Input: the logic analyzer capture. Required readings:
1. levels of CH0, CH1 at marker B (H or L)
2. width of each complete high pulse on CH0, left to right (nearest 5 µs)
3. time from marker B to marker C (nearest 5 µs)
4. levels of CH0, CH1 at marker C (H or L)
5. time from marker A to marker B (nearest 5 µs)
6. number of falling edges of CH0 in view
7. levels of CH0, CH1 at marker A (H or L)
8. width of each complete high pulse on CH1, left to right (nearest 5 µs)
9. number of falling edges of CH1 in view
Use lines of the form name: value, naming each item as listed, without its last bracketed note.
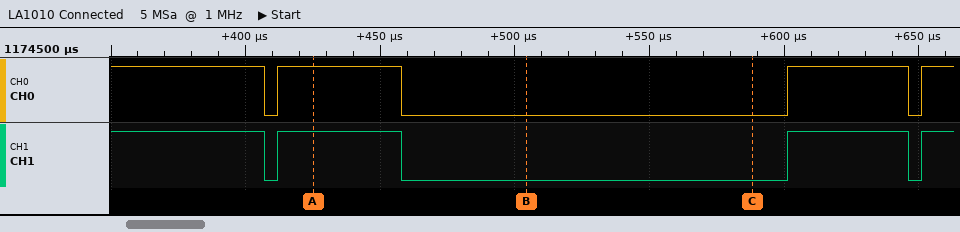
levels of CH0, CH1 at marker B: CH0=L, CH1=L
width of each complete high pulse on CH0, left to right: 45 µs, 45 µs
time from marker B to marker C: 85 µs
levels of CH0, CH1 at marker C: CH0=L, CH1=L
time from marker A to marker B: 80 µs
number of falling edges of CH0 in view: 3
levels of CH0, CH1 at marker A: CH0=H, CH1=H
width of each complete high pulse on CH1, left to right: 45 µs, 45 µs
number of falling edges of CH1 in view: 3
